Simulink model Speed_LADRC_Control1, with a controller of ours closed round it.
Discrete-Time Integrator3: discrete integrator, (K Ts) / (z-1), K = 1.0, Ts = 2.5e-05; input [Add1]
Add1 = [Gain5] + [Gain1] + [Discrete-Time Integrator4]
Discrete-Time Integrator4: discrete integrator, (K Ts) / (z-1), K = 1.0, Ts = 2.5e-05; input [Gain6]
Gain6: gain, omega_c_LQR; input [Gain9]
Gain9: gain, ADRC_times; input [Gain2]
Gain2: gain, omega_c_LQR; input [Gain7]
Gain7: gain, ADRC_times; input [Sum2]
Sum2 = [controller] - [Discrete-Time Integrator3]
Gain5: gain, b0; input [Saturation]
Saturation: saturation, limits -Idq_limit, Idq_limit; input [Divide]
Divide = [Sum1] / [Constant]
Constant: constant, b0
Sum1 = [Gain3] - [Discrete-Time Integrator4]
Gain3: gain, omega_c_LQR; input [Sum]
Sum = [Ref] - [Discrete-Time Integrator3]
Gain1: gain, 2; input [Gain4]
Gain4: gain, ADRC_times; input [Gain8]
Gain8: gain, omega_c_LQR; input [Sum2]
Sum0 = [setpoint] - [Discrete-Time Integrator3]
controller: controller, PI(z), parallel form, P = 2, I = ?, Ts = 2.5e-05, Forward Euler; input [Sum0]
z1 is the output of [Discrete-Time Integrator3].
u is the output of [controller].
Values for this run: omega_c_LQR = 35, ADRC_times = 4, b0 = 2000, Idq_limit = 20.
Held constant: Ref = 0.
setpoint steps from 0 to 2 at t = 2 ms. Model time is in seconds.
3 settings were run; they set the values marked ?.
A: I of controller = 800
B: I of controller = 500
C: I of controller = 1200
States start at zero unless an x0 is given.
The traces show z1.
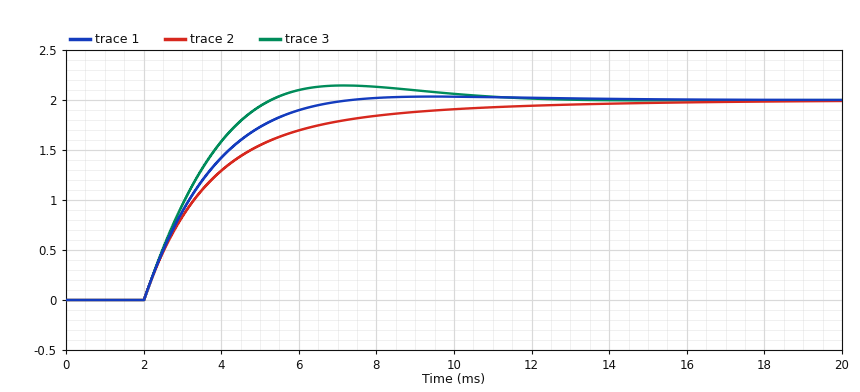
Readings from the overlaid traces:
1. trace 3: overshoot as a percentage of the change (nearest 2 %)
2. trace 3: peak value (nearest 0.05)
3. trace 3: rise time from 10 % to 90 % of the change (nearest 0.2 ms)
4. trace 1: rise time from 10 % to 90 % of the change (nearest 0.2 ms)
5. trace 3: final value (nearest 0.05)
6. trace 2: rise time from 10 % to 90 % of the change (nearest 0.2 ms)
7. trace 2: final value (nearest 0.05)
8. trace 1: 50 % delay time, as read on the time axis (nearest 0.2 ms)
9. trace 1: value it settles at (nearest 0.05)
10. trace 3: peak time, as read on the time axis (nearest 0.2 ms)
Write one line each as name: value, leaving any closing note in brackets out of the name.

trace 3: overshoot as a percentage of the change: 8 %
trace 3: peak value: 2.15
trace 3: rise time from 10 % to 90 % of the change: 2.4 ms
trace 1: rise time from 10 % to 90 % of the change: 3.2 ms
trace 3: final value: 2.00
trace 2: rise time from 10 % to 90 % of the change: 5.0 ms
trace 2: final value: 2.00
trace 1: 50 % delay time, as read on the time axis: 3.2 ms
trace 1: value it settles at: 2.00
trace 3: peak time, as read on the time axis: 7.2 ms
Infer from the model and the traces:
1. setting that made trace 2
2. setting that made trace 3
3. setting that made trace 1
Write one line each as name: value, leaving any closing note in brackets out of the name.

setting that made trace 2: B
setting that made trace 3: C
setting that made trace 1: A
